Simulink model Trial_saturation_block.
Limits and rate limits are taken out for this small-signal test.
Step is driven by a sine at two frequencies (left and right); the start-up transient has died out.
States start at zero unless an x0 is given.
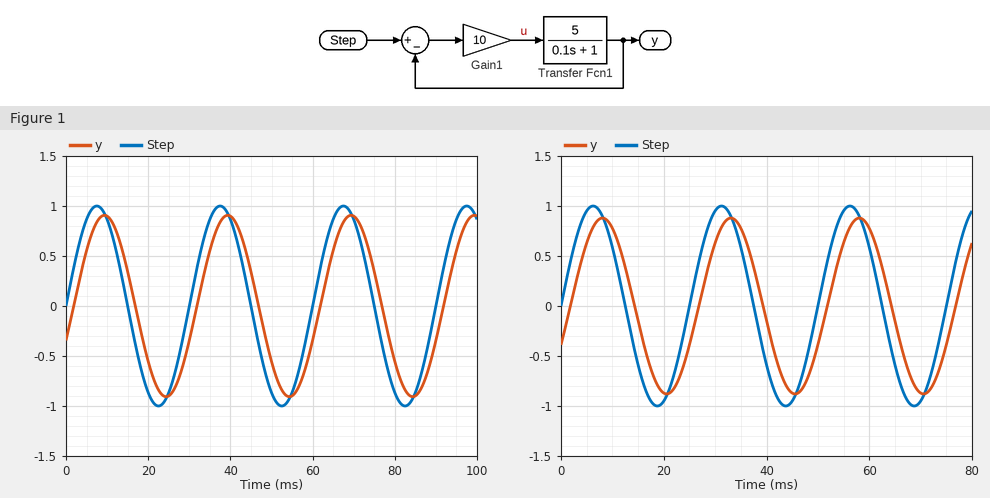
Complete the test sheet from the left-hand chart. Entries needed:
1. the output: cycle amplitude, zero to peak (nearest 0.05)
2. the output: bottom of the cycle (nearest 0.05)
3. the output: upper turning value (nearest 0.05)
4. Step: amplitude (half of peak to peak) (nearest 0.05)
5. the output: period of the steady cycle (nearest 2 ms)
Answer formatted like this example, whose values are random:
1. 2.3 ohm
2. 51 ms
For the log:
1. 0.90
2. -0.90
3. 0.90
4. 1.00
5. 30 ms
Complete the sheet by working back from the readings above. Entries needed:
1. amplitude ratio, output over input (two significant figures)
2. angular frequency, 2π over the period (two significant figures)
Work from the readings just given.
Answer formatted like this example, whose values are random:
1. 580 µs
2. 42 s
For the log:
1. 0.90
2. 0.21 rad/ms
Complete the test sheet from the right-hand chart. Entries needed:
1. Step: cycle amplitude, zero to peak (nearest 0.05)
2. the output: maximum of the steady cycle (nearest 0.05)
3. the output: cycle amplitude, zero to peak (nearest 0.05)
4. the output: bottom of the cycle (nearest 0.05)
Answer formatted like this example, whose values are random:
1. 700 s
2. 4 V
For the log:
1. 1.00
2. 0.90
3. 0.90
4. -0.90
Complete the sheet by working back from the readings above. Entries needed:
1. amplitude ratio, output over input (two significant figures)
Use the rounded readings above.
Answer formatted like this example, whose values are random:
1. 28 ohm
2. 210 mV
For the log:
1. 0.90
